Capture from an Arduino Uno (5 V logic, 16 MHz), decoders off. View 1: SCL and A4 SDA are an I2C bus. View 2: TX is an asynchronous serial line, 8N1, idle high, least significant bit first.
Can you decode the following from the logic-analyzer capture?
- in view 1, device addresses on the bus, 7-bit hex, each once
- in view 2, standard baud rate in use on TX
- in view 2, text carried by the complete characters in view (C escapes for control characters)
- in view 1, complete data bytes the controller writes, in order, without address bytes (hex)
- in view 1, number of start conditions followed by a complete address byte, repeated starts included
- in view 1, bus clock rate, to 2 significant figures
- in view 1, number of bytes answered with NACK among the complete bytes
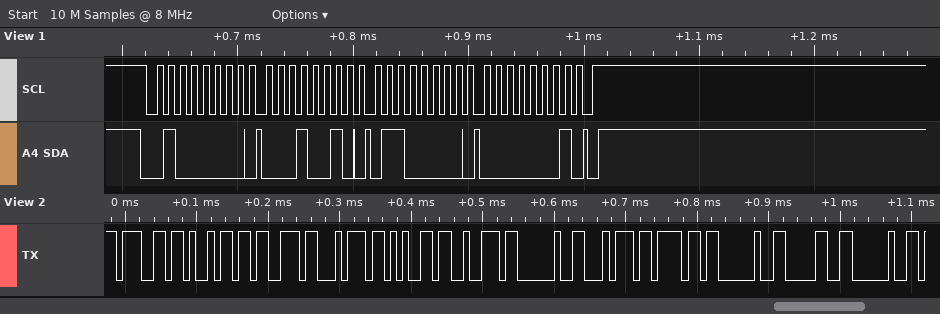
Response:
0x20
115200 baud
"gister to 0 "
12 60 01
1
100 kHz
0
